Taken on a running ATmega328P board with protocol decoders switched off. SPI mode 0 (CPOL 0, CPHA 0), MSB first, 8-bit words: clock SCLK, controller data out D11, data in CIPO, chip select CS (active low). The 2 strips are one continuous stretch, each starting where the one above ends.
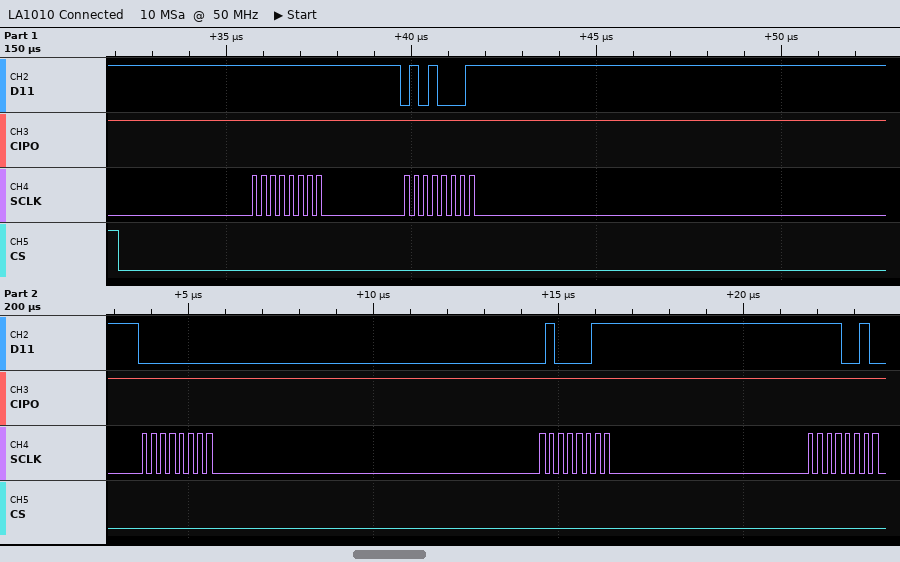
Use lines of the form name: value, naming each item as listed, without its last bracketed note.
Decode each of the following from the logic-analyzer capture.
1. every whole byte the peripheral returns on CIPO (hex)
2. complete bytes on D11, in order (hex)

every whole byte the peripheral returns on CIPO: 0xFF 0xFF 0xFF 0xFF 0xFF
complete bytes on D11, in order: 0xFF 0x51 0x00 0x43 0xF2
